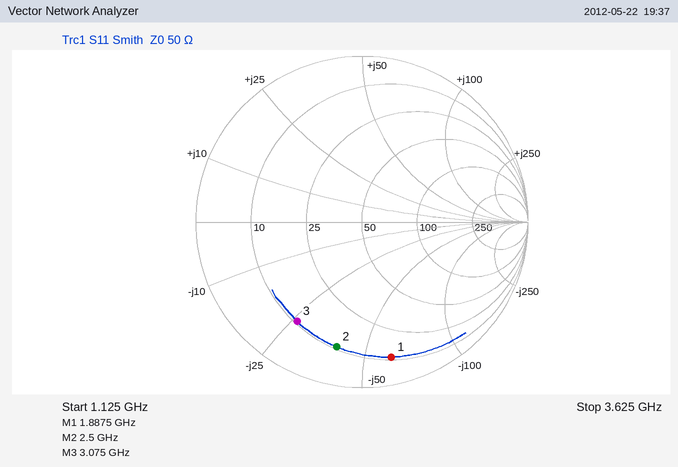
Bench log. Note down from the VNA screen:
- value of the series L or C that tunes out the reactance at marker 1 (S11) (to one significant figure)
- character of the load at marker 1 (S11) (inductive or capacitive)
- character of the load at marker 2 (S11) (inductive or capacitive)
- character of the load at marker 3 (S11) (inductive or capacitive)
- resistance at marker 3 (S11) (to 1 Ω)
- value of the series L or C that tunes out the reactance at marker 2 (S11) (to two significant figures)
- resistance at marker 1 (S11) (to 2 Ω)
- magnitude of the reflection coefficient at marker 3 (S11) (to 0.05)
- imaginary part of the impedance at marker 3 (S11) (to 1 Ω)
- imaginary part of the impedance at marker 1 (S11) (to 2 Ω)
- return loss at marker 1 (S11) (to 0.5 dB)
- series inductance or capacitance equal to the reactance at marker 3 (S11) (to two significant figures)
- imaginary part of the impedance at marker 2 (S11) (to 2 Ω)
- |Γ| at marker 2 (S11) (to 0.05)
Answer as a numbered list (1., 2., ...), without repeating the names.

1. 5 nH
2. capacitive
3. capacitive
4. capacitive
5. 11 Ω
6. 2.5 nH
7. 12 Ω
8. 0.70
9. -26 Ω
10. -60 Ω
11. 1.5 dB
12. 2.0 pF
13. -40 Ω
14. 0.75
